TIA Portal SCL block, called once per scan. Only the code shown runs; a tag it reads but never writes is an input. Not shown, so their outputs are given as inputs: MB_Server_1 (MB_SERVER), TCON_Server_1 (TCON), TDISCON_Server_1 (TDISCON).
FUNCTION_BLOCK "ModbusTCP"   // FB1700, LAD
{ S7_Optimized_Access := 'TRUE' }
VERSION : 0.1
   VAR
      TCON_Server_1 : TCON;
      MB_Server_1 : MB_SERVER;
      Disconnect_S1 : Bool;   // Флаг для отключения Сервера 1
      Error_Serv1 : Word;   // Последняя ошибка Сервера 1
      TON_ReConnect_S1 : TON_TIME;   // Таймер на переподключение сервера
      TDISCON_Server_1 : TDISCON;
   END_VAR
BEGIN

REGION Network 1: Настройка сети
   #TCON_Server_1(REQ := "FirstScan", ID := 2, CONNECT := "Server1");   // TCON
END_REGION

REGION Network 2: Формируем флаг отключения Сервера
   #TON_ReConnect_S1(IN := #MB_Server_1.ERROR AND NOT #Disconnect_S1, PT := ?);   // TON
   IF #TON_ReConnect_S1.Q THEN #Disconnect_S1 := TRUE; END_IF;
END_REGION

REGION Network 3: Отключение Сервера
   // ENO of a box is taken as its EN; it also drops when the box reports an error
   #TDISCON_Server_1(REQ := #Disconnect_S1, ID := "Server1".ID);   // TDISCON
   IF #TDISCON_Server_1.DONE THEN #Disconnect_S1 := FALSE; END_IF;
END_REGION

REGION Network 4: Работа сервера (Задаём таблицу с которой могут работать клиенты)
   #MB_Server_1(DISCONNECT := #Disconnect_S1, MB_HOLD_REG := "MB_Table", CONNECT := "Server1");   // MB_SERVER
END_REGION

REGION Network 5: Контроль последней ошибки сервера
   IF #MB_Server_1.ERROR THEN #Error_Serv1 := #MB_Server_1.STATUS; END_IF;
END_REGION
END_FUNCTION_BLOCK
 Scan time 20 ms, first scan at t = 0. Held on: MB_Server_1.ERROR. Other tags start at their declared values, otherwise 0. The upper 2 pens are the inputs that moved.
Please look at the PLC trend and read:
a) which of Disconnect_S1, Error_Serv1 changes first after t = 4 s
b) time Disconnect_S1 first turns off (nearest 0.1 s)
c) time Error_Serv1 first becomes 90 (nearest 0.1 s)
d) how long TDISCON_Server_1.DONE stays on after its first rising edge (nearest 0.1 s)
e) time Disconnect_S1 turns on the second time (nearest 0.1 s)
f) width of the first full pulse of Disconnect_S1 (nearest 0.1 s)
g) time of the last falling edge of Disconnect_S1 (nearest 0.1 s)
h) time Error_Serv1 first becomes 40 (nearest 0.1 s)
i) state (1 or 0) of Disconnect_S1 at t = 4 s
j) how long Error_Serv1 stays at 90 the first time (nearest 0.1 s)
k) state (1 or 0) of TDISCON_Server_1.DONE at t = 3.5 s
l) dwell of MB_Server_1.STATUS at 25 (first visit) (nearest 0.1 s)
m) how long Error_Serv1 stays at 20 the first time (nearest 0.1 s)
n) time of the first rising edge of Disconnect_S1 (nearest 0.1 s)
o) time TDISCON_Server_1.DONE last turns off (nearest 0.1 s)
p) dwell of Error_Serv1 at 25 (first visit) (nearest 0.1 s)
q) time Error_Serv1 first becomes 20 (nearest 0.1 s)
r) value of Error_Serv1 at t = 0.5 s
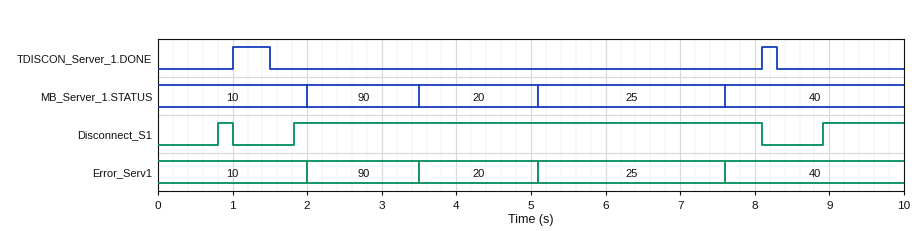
Error_Serv1
1.0 s
2.0 s
0.5 s
1.8 s
0.2 s
8.1 s
7.6 s
1
1.5 s
0
2.5 s
1.6 s
0.8 s
8.3 s
2.5 s
3.5 s
10
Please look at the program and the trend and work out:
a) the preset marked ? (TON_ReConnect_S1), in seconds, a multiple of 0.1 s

0.8 s
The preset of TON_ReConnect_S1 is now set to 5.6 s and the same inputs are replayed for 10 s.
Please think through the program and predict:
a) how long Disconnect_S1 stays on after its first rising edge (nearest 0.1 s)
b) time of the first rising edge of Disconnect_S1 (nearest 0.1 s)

2.5 s
5.6 s
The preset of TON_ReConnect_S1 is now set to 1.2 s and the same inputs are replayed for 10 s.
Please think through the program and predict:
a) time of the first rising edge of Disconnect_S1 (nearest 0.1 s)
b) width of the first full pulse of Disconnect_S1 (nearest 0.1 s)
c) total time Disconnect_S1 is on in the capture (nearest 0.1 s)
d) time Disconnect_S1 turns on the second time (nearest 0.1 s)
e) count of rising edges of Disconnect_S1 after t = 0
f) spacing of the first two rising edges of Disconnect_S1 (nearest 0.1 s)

1.5 s
6.6 s
7.3 s
9.3 s
2
7.8 s
